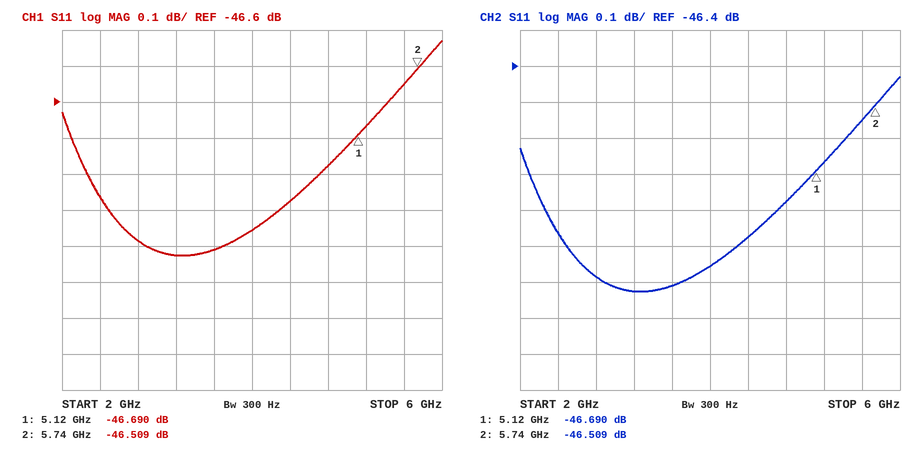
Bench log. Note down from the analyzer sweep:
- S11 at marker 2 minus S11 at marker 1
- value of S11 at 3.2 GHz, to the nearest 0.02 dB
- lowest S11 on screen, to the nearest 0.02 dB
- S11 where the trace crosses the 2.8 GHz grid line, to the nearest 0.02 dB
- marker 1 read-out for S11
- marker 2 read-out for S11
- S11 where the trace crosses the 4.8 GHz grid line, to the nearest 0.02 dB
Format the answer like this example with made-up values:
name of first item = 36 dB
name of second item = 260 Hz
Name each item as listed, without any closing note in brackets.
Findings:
S11 at marker 2 minus S11 at marker 1 = 0.181 dB
value of S11 at 3.2 GHz, to the nearest 0.02 dB = -47.02 dB
lowest S11 on screen, to the nearest 0.02 dB = -47.02 dB
S11 where the trace crosses the 2.8 GHz grid line, to the nearest 0.02 dB = -46.98 dB
marker 1 read-out for S11 = -46.690 dB
marker 2 read-out for S11 = -46.509 dB
S11 where the trace crosses the 4.8 GHz grid line, to the nearest 0.02 dB = -46.78 dB
